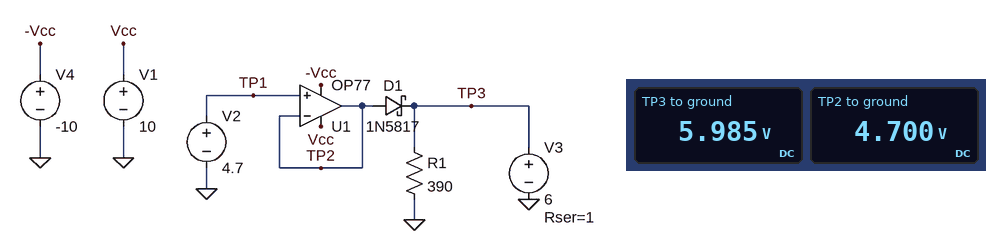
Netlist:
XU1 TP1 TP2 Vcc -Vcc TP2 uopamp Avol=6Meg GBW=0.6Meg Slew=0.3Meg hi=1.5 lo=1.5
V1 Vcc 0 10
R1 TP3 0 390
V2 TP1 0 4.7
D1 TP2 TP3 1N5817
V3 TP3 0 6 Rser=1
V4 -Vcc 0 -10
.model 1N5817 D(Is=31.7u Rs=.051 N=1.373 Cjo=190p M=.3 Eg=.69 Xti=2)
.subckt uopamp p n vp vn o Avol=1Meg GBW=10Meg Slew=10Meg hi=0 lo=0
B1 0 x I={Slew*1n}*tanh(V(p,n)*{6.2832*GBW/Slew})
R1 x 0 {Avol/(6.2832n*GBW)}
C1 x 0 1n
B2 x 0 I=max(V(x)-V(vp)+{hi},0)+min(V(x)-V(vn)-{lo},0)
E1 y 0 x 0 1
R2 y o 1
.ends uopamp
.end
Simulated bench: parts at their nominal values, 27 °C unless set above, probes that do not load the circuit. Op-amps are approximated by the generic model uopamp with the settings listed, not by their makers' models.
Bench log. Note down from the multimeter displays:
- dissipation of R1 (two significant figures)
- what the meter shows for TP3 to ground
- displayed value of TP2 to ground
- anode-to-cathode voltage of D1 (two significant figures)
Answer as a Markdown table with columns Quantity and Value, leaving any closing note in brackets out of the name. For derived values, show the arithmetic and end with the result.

| Quantity | Value |
|---|---|
| dissipation of R1 | (5.985 V)^2 / 390 Ω = 92 mW |
| what the meter shows for TP3 to ground | 5.985 V |
| displayed value of TP2 to ground | 4.700 V |
| anode-to-cathode voltage of D1 | 4.7 V - 5.985 V = -1.3 V |
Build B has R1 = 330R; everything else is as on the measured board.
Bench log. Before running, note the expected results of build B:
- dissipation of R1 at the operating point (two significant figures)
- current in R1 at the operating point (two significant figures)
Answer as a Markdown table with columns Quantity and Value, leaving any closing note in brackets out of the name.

| Quantity | Value |
|---|---|
| dissipation of R1 at the operating point | 110 mW |
| current in R1 at the operating point | 18 mA |
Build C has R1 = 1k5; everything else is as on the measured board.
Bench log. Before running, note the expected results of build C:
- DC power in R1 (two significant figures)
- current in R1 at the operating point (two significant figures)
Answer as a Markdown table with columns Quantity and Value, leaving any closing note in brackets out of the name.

| Quantity | Value |
|---|---|
| DC power in R1 | 24 mW |
| current in R1 at the operating point | 4.0 mA |
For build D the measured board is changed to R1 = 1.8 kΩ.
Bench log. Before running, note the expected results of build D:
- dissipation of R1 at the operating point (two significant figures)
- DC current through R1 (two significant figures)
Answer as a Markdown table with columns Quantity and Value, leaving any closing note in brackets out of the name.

| Quantity | Value |
|---|---|
| dissipation of R1 at the operating point | 20 mW |
| DC current through R1 | 3.3 mA |
